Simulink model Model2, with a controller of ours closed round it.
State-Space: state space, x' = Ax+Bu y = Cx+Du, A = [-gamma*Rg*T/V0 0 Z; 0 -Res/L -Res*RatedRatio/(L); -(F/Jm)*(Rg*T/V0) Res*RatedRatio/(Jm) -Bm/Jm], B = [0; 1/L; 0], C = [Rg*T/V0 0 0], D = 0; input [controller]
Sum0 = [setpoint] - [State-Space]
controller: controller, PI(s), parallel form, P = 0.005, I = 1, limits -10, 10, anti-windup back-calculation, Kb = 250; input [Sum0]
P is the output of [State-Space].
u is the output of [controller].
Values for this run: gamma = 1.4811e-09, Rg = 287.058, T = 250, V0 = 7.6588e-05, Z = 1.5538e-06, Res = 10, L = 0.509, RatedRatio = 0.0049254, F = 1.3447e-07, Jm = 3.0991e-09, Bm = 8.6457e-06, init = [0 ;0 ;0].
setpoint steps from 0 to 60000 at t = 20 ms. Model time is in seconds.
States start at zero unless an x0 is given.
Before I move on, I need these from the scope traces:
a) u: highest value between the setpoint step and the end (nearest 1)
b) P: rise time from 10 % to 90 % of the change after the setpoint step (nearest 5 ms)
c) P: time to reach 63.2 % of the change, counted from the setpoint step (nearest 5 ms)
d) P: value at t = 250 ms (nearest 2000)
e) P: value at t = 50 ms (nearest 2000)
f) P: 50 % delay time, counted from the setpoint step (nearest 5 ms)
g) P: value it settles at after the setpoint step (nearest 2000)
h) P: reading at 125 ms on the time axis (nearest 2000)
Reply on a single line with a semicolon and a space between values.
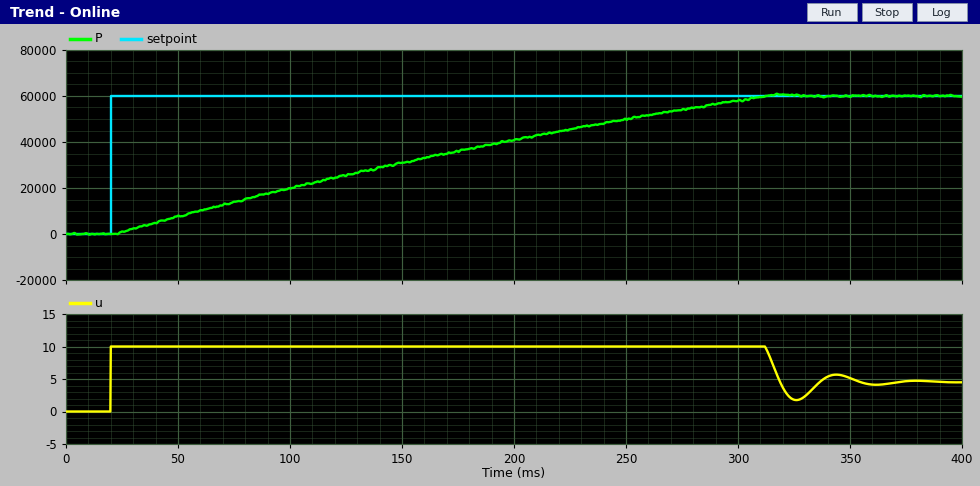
10; 230 ms; 165 ms; 50000; 8000; 125 ms; 60000; 26000
